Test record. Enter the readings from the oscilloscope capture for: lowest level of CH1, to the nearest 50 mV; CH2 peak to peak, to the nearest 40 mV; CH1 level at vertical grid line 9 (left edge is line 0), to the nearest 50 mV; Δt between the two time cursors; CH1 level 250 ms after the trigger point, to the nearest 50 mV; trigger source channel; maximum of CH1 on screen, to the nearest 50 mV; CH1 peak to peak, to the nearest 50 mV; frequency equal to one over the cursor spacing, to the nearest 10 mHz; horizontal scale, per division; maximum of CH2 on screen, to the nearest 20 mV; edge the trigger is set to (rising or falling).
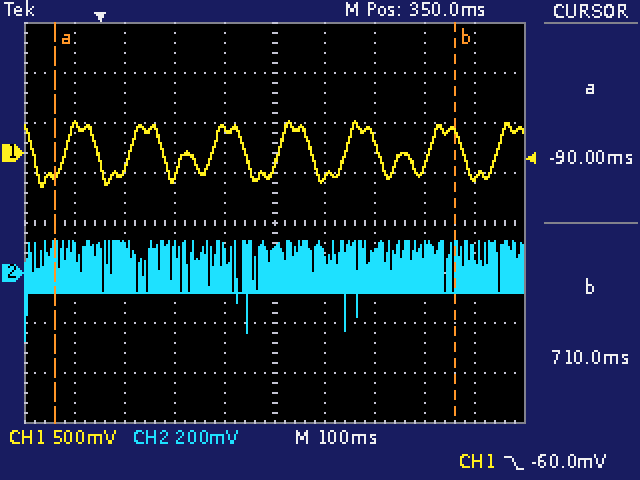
-350 mV
400 mV
-250 mV
800 ms
250 mV
CH1
300 mV
650 mV
1.25 Hz
100 ms
120 mV
falling
